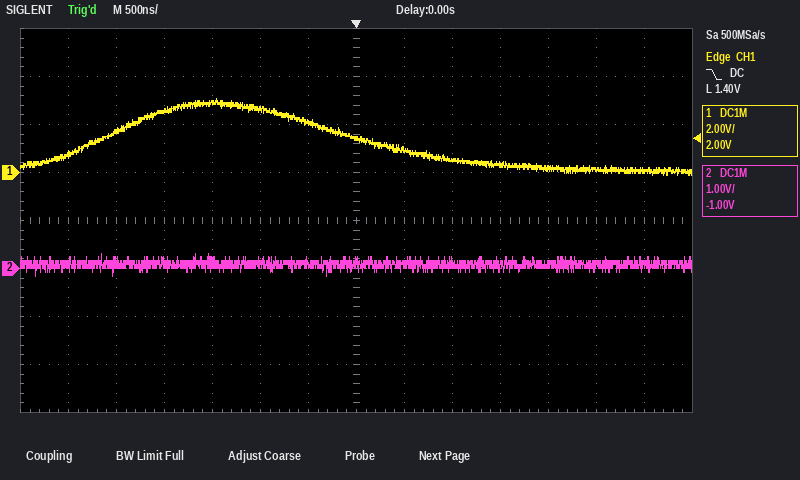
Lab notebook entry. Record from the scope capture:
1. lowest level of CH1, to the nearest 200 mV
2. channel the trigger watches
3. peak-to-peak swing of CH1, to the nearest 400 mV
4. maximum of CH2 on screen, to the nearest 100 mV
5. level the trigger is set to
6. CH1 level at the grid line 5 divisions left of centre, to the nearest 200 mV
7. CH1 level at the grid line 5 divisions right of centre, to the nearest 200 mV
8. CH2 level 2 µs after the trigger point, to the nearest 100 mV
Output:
-200 mV
CH1
3.2 V
300 mV
1.40 V
1.8 V
200 mV
100 mV
